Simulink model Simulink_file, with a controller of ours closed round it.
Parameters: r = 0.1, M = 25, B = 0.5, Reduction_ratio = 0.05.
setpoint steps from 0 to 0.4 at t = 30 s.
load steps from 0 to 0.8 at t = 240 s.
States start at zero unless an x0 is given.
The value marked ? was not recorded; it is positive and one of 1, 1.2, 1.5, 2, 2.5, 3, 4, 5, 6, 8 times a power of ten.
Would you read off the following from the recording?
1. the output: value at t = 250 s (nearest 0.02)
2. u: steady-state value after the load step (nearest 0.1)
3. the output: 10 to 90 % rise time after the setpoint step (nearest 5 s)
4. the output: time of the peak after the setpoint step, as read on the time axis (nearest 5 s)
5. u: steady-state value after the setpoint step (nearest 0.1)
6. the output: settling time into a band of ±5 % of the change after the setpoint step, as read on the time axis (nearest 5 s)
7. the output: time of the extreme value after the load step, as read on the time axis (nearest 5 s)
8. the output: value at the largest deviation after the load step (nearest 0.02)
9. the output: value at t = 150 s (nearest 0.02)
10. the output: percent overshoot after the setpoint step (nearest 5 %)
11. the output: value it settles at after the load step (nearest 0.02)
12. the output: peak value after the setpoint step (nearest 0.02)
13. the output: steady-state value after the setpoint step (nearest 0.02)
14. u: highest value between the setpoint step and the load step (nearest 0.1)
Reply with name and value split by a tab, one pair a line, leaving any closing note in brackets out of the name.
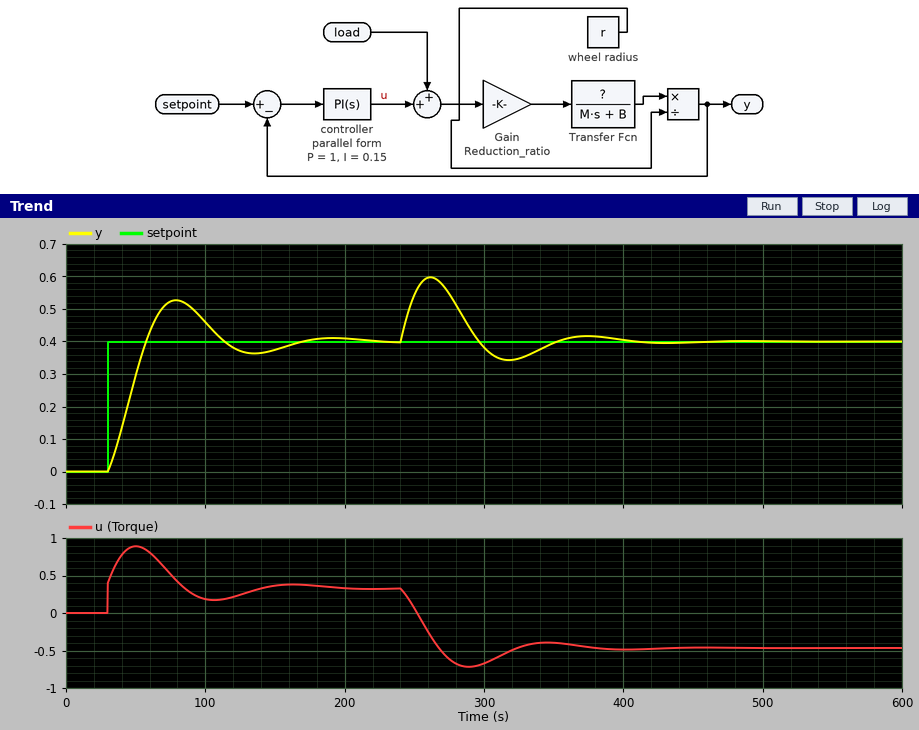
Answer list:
the output: value at t = 250 s	0.54
u: steady-state value after the load step	-0.5
the output: 10 to 90 % rise time after the setpoint step	20 s
the output: time of the peak after the setpoint step, as read on the time axis	80 s
u: steady-state value after the setpoint step	0.3
the output: settling time into a band of ±5 % of the change after the setpoint step, as read on the time axis	155 s
the output: time of the extreme value after the load step, as read on the time axis	260 s
the output: value at the largest deviation after the load step	0.60
the output: value at t = 150 s	0.38
the output: percent overshoot after the setpoint step	30 %
the output: value it settles at after the load step	0.40
the output: peak value after the setpoint step	0.52
the output: steady-state value after the setpoint step	0.40
u: highest value between the setpoint step and the load step	0.9
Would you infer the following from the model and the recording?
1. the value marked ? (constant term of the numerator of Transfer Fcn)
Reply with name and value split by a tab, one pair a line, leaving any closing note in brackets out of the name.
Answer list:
the value marked ?	1.2
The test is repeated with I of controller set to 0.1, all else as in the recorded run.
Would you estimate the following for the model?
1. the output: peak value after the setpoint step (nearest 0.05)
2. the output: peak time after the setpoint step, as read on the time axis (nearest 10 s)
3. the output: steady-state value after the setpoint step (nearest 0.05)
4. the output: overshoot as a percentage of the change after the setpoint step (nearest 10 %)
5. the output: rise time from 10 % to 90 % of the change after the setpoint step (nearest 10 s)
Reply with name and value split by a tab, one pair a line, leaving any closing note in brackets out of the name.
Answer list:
the output: peak value after the setpoint step	0.50
the output: peak time after the setpoint step, as read on the time axis	90 s
the output: steady-state value after the setpoint step	0.40
the output: overshoot as a percentage of the change after the setpoint step	20 %
the output: rise time from 10 % to 90 % of the change after the setpoint step	30 s
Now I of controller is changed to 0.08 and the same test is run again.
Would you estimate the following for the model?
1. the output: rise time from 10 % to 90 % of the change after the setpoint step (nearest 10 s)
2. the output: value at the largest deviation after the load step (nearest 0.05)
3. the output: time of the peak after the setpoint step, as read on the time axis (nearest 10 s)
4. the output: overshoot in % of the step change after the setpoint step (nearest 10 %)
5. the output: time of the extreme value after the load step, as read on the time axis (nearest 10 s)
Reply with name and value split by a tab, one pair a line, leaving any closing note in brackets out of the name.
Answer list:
the output: rise time from 10 % to 90 % of the change after the setpoint step	30 s
the output: value at the largest deviation after the load step	0.65
the output: time of the peak after the setpoint step, as read on the time axis	100 s
the output: overshoot in % of the step change after the setpoint step	20 %
the output: time of the extreme value after the load step, as read on the time axis	270 s
